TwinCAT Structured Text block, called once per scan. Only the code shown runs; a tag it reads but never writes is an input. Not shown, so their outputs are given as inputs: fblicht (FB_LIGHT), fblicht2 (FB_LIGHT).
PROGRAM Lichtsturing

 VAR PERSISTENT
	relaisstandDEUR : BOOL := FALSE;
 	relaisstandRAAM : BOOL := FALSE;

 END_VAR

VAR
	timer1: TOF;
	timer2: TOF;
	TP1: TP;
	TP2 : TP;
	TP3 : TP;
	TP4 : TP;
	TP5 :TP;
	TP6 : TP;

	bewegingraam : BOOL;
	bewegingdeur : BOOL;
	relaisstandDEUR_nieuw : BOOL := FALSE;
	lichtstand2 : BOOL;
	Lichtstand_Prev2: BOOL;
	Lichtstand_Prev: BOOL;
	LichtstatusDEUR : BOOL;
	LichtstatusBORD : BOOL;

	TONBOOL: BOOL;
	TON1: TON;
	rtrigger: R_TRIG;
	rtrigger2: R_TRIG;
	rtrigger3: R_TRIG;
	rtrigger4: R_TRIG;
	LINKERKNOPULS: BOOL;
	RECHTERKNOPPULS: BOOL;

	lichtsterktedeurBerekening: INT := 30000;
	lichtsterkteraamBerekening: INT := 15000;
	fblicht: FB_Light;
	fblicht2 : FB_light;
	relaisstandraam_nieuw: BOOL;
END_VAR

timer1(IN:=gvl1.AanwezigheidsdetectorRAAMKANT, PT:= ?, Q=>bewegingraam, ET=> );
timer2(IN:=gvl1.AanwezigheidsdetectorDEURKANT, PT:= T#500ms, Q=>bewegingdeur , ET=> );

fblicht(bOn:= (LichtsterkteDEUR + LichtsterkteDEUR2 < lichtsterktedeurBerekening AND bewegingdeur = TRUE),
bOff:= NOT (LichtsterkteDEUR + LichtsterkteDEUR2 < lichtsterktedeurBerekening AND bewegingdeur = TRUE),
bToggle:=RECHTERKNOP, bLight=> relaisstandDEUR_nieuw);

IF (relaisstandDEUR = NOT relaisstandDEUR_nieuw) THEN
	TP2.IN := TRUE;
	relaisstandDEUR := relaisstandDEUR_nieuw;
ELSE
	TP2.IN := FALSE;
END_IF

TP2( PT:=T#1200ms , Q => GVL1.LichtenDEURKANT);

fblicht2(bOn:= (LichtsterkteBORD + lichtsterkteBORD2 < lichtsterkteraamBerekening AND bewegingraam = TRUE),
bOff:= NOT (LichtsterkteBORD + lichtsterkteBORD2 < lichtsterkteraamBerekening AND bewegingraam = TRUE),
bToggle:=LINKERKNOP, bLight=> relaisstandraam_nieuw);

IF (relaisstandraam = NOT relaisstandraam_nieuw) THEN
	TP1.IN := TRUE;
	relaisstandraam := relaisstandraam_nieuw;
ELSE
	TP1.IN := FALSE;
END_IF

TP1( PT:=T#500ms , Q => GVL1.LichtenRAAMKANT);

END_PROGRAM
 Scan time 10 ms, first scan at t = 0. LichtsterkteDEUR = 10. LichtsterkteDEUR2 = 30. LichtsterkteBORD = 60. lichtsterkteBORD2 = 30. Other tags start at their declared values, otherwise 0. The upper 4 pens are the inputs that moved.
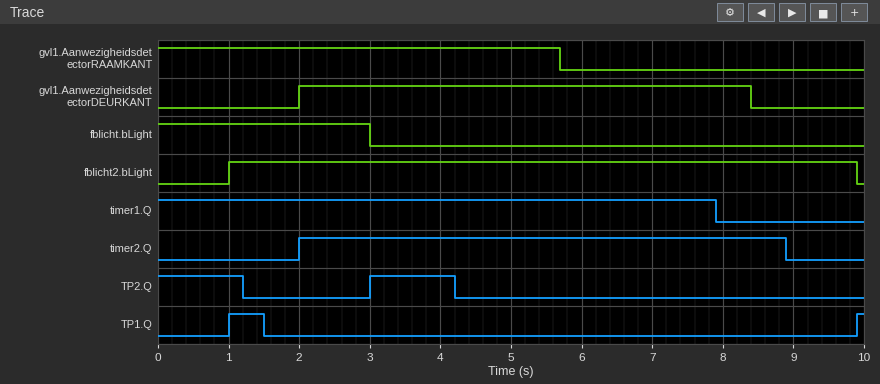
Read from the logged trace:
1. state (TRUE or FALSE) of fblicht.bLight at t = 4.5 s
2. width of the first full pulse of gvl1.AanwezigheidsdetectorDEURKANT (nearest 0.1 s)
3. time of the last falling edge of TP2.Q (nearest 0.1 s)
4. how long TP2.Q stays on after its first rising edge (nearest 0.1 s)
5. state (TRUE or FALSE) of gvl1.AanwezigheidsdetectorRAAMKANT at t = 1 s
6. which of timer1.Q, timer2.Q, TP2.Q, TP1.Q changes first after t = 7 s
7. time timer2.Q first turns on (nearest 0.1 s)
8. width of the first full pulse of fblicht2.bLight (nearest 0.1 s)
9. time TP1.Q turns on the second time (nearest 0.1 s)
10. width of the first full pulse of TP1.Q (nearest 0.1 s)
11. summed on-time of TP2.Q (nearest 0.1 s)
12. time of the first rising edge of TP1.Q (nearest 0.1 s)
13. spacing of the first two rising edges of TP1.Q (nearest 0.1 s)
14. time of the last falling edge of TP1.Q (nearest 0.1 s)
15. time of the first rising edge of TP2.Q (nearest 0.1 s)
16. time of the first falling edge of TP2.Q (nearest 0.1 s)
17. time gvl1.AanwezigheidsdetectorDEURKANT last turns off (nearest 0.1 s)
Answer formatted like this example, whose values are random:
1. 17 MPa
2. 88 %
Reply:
1. FALSE
2. 6.4 s
3. 4.2 s
4. 1.2 s
5. TRUE
6. timer1.Q
7. 2.0 s
8. 8.9 s
9. 9.9 s
10. 0.5 s
11. 2.4 s
12. 1.0 s
13. 8.9 s
14. 1.5 s
15. 3.0 s
16. 1.2 s
17. 8.4 s
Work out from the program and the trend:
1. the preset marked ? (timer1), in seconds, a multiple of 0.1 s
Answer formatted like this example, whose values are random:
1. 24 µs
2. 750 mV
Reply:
1. 2.2 s
